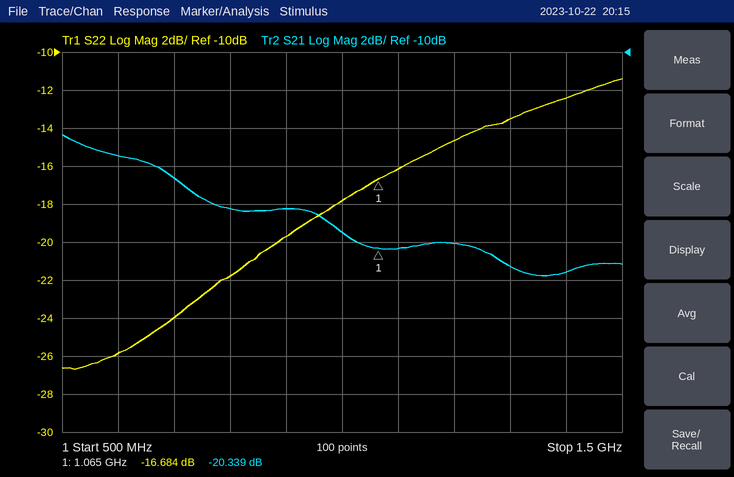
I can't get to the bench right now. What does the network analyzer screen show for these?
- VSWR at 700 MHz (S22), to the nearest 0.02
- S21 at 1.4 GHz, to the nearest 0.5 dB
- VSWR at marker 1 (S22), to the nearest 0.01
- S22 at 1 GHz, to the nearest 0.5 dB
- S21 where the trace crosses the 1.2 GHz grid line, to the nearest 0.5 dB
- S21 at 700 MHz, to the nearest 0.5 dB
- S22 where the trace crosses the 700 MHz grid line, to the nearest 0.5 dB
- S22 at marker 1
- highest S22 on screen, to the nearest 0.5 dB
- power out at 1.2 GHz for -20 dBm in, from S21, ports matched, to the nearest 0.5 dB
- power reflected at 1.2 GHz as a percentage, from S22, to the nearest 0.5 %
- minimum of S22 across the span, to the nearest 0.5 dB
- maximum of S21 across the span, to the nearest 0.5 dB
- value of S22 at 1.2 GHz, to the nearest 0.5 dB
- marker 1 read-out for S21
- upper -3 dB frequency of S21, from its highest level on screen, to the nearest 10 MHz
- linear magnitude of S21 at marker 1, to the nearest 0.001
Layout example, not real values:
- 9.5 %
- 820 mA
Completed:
- 1.14
- -21.5 dB
- 1.34
- -18.0 dB
- -20.0 dB
- -16.5 dB
- -24.0 dB
- -16.684 dB
- -11.5 dB
- -40.0 dBm
- 3.5 %
- -26.5 dB
- -14.5 dB
- -14.5 dB
- -20.339 dB
- 730 MHz
- 0.096
